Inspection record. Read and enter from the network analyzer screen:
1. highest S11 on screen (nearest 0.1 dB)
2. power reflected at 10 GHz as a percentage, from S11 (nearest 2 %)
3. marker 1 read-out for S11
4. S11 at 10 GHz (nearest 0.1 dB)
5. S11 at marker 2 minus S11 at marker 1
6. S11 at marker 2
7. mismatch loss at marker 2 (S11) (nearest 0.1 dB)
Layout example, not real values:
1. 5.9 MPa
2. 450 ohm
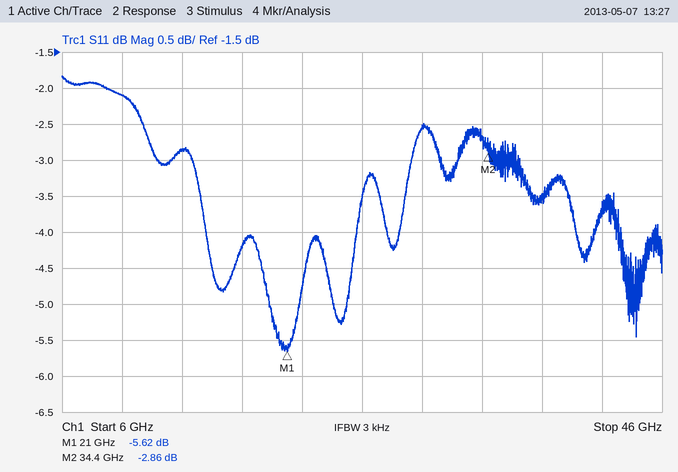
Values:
1. -1.8 dB
2. 62 %
3. -5.62 dB
4. -2.1 dB
5. 2.76 dB
6. -2.86 dB
7. 3.2 dB
